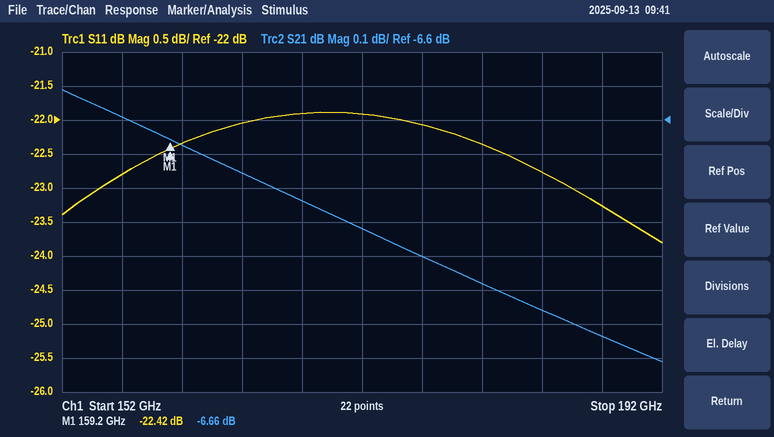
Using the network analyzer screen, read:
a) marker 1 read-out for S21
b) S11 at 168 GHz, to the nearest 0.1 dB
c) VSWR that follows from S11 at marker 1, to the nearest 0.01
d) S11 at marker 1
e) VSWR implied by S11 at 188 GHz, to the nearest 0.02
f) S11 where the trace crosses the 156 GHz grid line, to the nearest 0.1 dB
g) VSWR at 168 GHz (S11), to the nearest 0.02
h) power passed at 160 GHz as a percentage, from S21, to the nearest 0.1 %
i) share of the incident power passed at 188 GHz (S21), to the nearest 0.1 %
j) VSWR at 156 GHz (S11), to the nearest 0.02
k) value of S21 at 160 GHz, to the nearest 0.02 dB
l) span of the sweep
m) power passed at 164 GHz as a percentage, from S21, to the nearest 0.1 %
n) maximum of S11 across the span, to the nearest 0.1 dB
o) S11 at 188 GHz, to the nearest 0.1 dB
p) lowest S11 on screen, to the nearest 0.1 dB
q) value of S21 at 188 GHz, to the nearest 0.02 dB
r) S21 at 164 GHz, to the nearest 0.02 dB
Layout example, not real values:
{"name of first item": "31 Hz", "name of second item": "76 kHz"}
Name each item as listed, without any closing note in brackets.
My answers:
{"marker 1 read-out for S21": "-6.66 dB", "S11 at 168 GHz, to the nearest 0.1 dB": "-21.9 dB", "VSWR that follows from S11 at marker 1, to the nearest 0.01": "1.16", "S11 at marker 1": "-22.42 dB", "VSWR implied by S11 at 188 GHz, to the nearest 0.02": "1.14", "S11 where the trace crosses the 156 GHz grid line, to the nearest 0.1 dB": "-22.8 dB", "VSWR at 168 GHz (S11), to the nearest 0.02": "1.18", "power passed at 160 GHz as a percentage, from S21, to the nearest 0.1 %": "21.5 %", "share of the incident power passed at 188 GHz (S21), to the nearest 0.1 %": "18.9 %", "VSWR at 156 GHz (S11), to the nearest 0.02": "1.16", "value of S21 at 160 GHz, to the nearest 0.02 dB": "-6.68 dB", "span of the sweep": "40 GHz", "power passed at 164 GHz as a percentage, from S21, to the nearest 0.1 %": "21.1 %", "maximum of S11 across the span, to the nearest 0.1 dB": "-21.9 dB", "S11 at 188 GHz, to the nearest 0.1 dB": "-23.3 dB", "lowest S11 on screen, to the nearest 0.1 dB": "-23.8 dB", "value of S21 at 188 GHz, to the nearest 0.02 dB": "-7.24 dB", "S21 at 164 GHz, to the nearest 0.02 dB": "-6.76 dB"}
